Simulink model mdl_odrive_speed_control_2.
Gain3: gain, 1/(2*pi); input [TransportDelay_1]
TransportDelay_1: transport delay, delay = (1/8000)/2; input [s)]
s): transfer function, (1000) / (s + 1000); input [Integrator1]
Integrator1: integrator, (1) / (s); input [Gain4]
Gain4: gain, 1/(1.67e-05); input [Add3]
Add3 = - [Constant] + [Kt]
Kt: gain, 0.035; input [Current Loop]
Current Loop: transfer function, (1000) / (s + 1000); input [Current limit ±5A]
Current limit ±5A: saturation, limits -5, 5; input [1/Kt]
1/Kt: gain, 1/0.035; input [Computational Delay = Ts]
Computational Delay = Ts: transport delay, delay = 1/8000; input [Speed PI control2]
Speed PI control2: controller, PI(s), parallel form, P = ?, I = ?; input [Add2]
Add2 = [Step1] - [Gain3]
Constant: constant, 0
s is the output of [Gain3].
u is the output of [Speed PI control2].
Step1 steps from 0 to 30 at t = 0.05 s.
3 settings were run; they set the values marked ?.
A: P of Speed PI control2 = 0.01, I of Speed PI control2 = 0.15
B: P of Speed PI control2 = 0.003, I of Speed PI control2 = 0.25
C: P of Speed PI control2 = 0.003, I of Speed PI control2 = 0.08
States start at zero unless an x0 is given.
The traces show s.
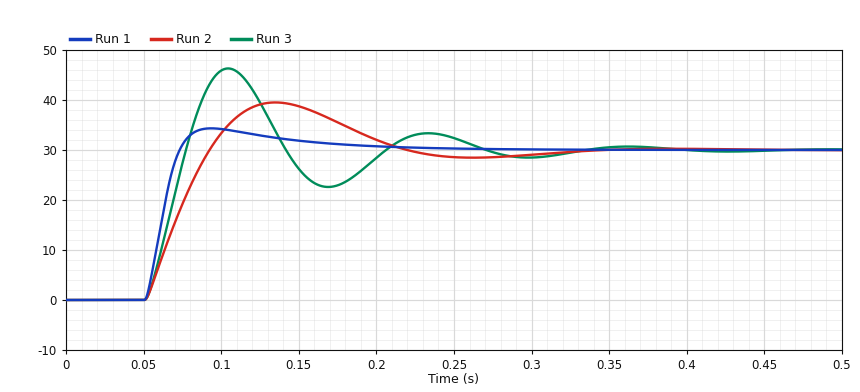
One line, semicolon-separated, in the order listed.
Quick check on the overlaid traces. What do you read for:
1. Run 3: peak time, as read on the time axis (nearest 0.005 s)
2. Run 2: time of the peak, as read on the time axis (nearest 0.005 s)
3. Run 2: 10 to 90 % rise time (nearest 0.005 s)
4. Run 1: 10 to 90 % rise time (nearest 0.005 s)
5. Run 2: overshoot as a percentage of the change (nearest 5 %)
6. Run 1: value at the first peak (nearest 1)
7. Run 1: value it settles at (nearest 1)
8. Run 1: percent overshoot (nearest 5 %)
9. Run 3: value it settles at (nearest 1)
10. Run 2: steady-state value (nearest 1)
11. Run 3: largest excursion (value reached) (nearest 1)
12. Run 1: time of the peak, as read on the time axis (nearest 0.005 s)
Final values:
0.105 s; 0.135 s; 0.030 s; 0.015 s; 30 %; 34; 30; 15 %; 30; 30; 46; 0.095 s
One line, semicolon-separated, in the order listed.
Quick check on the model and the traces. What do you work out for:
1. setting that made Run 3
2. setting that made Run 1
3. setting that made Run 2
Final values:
B; A; C
